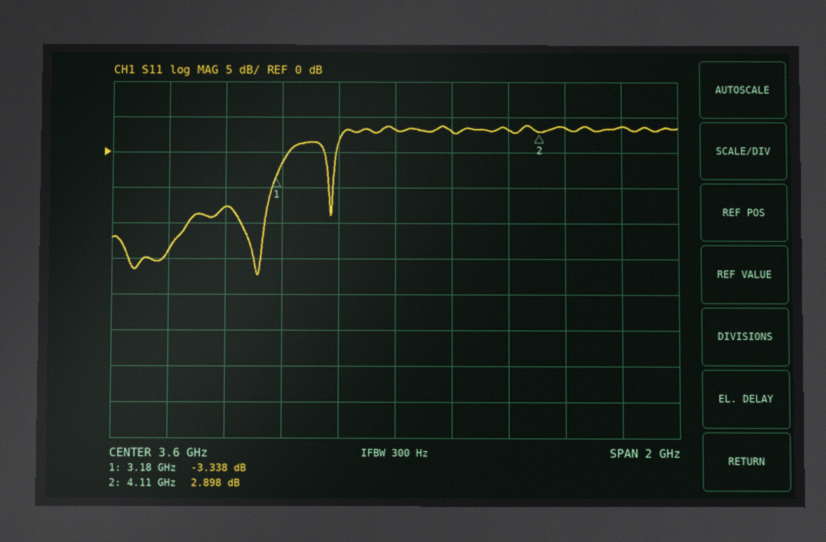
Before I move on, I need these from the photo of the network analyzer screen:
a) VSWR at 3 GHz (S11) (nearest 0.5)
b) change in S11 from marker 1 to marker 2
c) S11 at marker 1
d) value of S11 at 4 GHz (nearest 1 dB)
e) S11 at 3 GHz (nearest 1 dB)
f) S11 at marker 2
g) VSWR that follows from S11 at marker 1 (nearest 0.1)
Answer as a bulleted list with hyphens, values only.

- 2.5
- 6.236 dB
- -3.338 dB
- 3 dB
- -8 dB
- 2.898 dB
- 5.3
